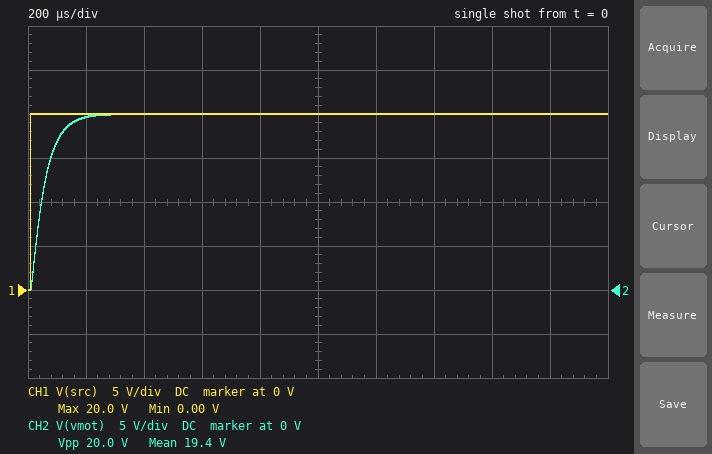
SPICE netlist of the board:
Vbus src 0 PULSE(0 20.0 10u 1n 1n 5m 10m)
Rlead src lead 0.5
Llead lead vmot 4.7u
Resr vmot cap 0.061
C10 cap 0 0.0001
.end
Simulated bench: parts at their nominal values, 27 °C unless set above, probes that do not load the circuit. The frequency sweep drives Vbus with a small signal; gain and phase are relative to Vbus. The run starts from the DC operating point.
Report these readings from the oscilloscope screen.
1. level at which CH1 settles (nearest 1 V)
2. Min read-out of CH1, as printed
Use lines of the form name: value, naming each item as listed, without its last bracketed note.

level at which CH1 settles: 20 V
Min read-out of CH1, as printed: 0.00 V
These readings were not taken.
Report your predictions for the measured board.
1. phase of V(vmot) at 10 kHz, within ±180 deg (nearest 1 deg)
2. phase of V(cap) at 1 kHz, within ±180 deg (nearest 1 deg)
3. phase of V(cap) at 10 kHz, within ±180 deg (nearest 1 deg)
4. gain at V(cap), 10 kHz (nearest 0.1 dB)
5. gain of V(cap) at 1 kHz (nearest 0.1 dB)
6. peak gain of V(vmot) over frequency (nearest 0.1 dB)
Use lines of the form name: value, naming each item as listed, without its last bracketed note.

phase of V(vmot) at 10 kHz, within ±180 deg: -83 deg
phase of V(cap) at 1 kHz, within ±180 deg: -20 deg
phase of V(cap) at 10 kHz, within ±180 deg: -104 deg
gain at V(cap), 10 kHz: -11.2 dB
gain of V(cap) at 1 kHz: -0.4 dB
peak gain of V(vmot) over frequency: 0 dB
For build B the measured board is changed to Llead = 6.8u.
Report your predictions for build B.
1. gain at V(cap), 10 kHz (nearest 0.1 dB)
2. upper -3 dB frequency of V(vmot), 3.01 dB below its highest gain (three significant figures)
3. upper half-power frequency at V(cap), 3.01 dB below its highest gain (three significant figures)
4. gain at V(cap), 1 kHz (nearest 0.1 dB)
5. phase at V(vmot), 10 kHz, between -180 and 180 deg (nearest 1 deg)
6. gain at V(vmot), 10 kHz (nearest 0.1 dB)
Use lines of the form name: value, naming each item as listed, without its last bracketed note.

gain at V(cap), 10 kHz: -11.8 dB
upper -3 dB frequency of V(vmot), 3.01 dB below its highest gain: 3.60 kHz
upper half-power frequency at V(cap), 3.01 dB below its highest gain: 3.54 kHz
gain at V(cap), 1 kHz: -0.3 dB
phase at V(vmot), 10 kHz, between -180 and 180 deg: -95 deg
gain at V(vmot), 10 kHz: -11.2 dB
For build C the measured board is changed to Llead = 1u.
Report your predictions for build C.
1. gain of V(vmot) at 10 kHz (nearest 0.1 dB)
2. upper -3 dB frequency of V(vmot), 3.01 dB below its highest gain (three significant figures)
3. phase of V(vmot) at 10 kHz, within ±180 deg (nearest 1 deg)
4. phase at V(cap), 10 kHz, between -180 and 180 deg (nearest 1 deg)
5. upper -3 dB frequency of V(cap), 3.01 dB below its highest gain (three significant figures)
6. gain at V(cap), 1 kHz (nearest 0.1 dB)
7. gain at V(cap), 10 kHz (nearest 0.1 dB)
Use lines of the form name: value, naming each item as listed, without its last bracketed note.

gain of V(vmot) at 10 kHz: -10.5 dB
upper -3 dB frequency of V(vmot), 3.01 dB below its highest gain: 2.97 kHz
phase of V(vmot) at 10 kHz, within ±180 deg: -59 deg
phase at V(cap), 10 kHz, between -180 and 180 deg: -80 deg
upper -3 dB frequency of V(cap), 3.01 dB below its highest gain: 2.93 kHz
gain at V(cap), 1 kHz: -0.5 dB
gain at V(cap), 10 kHz: -11.1 dB
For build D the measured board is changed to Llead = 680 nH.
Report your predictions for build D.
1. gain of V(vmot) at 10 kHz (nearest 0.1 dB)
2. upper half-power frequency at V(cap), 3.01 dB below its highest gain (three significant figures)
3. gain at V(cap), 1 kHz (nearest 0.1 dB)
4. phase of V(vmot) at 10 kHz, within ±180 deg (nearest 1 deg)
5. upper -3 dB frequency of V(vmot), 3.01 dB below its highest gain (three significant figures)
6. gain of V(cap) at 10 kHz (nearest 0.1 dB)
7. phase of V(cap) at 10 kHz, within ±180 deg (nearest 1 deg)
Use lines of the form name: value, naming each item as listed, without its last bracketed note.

gain of V(vmot) at 10 kHz: -10.5 dB
upper half-power frequency at V(cap), 3.01 dB below its highest gain: 2.90 kHz
gain at V(cap), 1 kHz: -0.5 dB
phase of V(vmot) at 10 kHz, within ±180 deg: -57 deg
upper -3 dB frequency of V(vmot), 3.01 dB below its highest gain: 2.94 kHz
gain of V(cap) at 10 kHz: -11.1 dB
phase of V(cap) at 10 kHz, within ±180 deg: -78 deg
